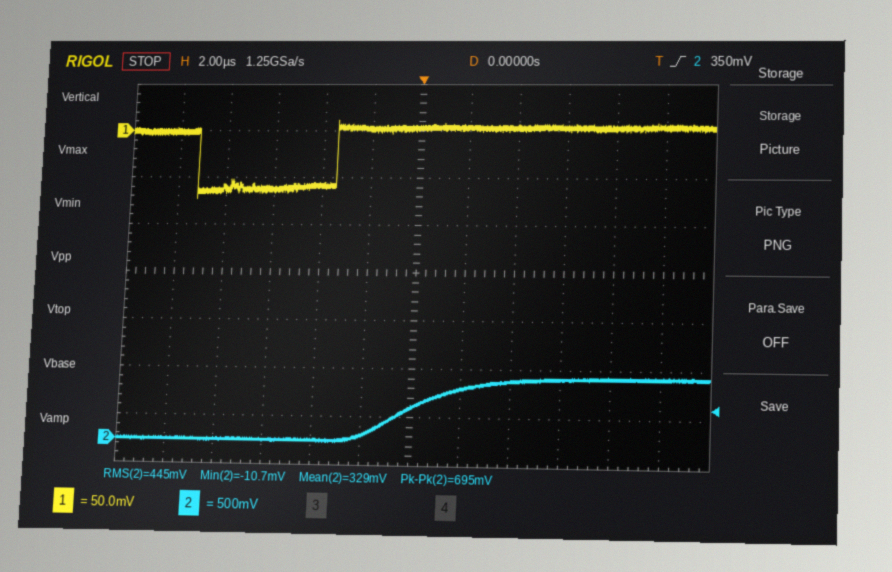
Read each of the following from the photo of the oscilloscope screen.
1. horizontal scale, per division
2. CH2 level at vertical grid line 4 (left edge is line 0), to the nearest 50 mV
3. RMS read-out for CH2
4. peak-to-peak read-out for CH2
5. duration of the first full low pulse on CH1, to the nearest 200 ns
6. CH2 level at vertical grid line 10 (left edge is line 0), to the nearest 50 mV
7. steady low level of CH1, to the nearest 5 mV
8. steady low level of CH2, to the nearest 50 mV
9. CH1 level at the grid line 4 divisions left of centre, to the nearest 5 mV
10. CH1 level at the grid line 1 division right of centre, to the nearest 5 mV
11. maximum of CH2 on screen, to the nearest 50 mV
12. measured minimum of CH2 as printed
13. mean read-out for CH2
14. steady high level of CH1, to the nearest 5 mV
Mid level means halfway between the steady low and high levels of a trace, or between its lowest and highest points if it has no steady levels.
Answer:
2 µs
0 mV
445 mV
695 mV
5.8 µs
650 mV
-60 mV
0 mV
-60 mV
5 mV
700 mV
-10.7 mV
329 mV
5 mV
